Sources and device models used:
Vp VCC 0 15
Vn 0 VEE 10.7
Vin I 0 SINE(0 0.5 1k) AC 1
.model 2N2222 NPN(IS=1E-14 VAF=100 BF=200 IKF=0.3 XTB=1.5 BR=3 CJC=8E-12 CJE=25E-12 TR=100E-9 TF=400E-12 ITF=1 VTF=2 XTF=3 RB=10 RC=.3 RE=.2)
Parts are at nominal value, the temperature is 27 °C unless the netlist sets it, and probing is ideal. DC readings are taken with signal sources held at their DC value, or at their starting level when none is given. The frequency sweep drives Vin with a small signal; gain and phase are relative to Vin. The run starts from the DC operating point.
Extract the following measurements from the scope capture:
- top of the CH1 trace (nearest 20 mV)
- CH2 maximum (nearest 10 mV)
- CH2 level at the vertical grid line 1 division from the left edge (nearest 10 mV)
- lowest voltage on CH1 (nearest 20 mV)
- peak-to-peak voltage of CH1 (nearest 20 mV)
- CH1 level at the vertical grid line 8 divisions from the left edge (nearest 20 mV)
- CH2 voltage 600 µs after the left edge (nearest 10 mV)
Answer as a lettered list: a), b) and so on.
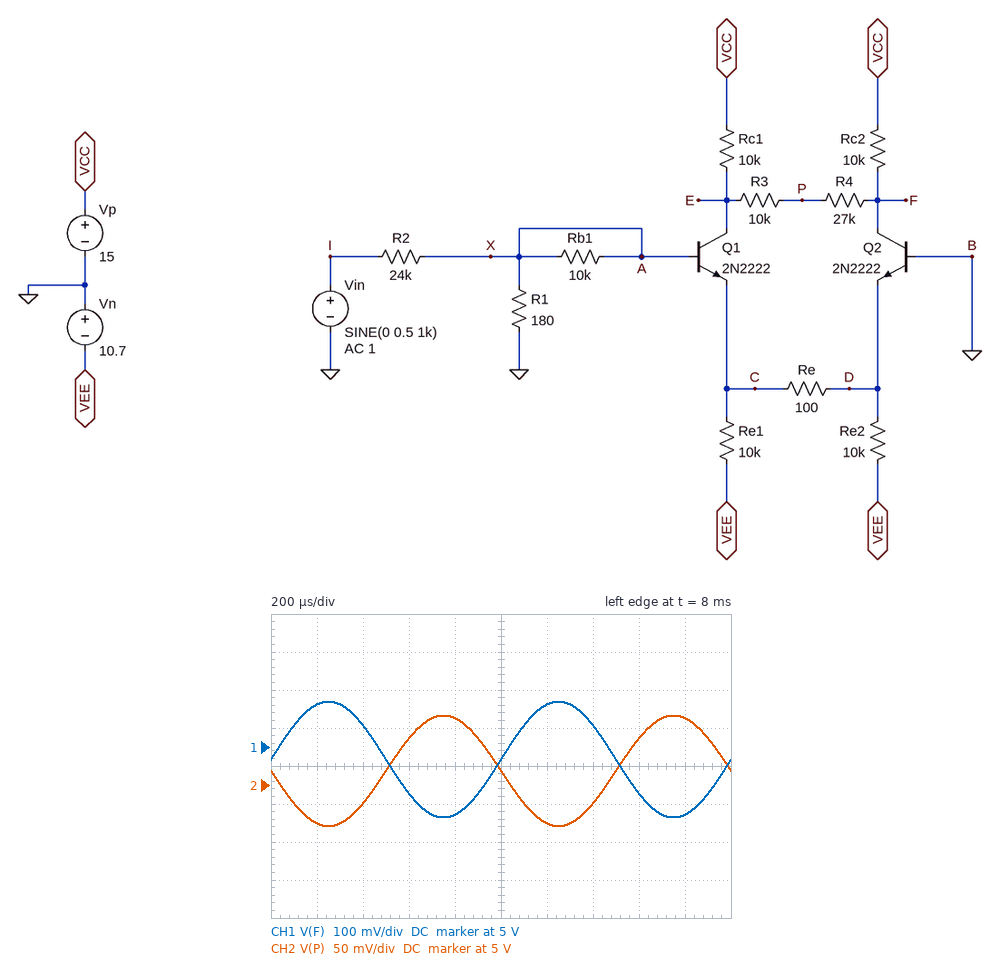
a) 5.12 V
b) 5.09 V
c) 4.95 V
d) 4.82 V
e) 300 mV
f) 4.88 V
g) 5.06 V
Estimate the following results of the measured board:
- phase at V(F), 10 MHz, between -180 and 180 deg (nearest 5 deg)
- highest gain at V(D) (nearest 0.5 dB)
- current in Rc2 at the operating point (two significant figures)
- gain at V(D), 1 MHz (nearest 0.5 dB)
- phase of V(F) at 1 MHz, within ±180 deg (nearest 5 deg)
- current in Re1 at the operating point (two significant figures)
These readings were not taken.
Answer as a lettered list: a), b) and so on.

a) -80 deg
b) -57.5 dB
c) 1.0 mA
d) -58.0 dB
e) -20 deg
f) 1.0 mA
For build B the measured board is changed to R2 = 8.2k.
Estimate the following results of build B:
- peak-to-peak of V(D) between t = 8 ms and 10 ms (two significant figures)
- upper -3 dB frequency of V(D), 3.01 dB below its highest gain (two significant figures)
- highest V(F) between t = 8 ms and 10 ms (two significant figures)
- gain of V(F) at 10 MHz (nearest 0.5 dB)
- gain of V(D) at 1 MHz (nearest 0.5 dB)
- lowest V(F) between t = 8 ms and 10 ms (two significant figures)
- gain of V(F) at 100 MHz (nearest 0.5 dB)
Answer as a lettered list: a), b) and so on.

a) 3.8 mV
b) 4.2 MHz
c) 5.4 V
d) -13.0 dB
e) -49.0 dB
f) 4.5 V
g) -35.0 dB
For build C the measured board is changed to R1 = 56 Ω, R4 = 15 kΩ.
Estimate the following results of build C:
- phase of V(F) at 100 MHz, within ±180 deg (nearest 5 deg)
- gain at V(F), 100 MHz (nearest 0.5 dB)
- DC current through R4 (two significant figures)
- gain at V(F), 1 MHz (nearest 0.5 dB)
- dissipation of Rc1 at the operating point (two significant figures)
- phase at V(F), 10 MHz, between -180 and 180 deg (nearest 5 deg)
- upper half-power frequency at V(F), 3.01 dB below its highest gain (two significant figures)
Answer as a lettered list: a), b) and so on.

a) -120 deg
b) -50.0 dB
c) 760 nA
d) -22.0 dB
e) 10 mW
f) -70 deg
g) 4.7 MHz
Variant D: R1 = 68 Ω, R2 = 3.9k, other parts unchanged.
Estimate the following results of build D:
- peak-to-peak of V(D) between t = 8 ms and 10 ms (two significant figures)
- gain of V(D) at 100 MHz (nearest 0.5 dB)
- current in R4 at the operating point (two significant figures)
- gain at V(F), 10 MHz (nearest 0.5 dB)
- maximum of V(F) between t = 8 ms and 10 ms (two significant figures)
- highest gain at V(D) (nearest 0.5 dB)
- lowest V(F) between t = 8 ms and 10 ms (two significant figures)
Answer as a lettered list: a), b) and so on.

a) 3.0 mV
b) -53.5 dB
c) 720 nA
d) -12.0 dB
e) 5.3 V
f) -50.5 dB
g) 4.6 V
